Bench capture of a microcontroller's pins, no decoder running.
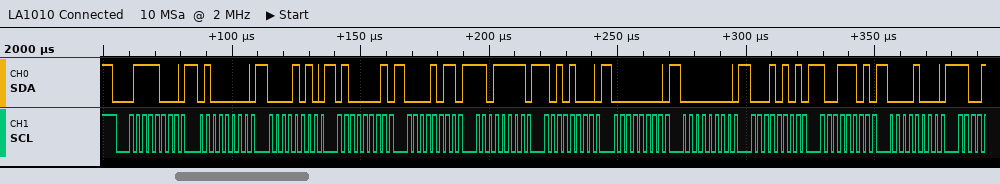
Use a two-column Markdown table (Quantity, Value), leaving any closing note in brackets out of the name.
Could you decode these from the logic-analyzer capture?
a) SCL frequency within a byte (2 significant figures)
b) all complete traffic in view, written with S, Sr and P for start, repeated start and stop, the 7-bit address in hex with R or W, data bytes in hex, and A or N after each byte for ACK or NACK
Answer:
| Quantity | Value |
|---|---|
| SCL frequency within a byte | 400 kHz |
| all complete traffic in view, written with S, Sr and P for start, repeated start and stop, the 7-bit address in hex with R or W, data bytes in hex, and A or N after each byte for ACK or NACK | S 3CW A 40 A 0A A 41 A 0B A DF A A8 A 00 A 00 A 15 A 9D A 08 A |
